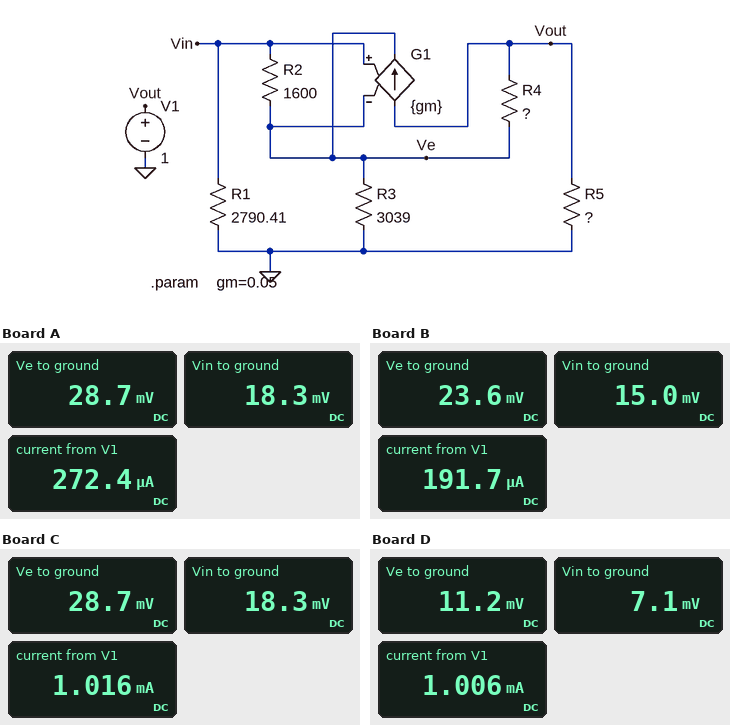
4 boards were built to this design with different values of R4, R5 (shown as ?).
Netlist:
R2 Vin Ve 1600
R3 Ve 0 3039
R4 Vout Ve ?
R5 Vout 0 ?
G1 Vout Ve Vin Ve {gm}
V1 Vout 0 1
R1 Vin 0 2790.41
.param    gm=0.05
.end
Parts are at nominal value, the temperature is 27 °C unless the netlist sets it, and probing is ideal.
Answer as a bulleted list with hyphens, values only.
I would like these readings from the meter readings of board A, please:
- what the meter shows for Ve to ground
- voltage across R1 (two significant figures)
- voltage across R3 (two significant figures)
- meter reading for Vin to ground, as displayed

- 28.7 mV
- 18 mV
- 29 mV
- 18.3 mV
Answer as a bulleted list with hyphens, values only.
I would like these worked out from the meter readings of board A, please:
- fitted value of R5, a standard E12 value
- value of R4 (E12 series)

- 3.9 kΩ
- 1.8 kΩ
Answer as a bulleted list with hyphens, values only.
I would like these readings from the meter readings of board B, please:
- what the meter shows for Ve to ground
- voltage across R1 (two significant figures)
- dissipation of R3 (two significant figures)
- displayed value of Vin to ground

- 23.6 mV
- 15 mV
- 180 nW
- 15.0 mV
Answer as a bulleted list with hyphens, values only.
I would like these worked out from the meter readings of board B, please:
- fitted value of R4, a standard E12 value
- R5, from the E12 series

- 2.2 kΩ
- 5.6 kΩ
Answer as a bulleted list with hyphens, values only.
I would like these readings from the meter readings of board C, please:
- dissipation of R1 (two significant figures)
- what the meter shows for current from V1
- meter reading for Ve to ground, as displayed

- 120 nW
- 1.016 mA
- 28.7 mV
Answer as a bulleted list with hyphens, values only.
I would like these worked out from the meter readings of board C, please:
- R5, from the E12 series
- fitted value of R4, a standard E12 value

- 1 kΩ
- 1.8 kΩ
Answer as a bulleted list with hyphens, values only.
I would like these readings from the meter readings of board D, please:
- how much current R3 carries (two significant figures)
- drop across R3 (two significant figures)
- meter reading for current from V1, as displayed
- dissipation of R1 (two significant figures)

- 3.7 µA
- 11 mV
- 1.006 mA
- 18 nW
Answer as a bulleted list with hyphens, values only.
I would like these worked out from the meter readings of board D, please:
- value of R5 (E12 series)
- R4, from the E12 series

- 1 kΩ
- 4.7 kΩ
